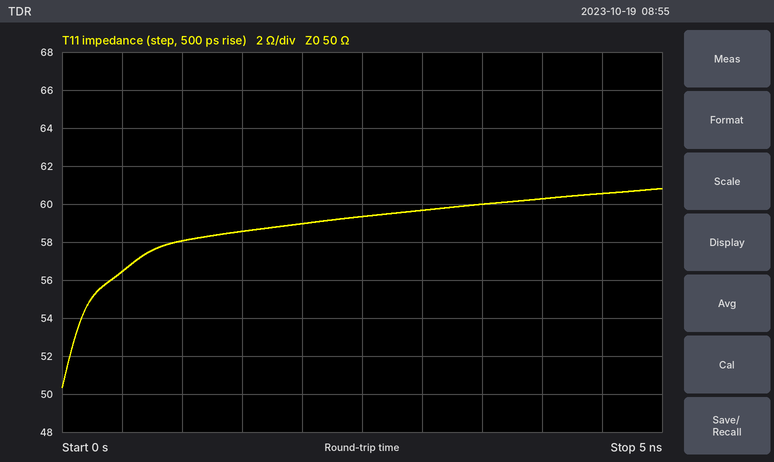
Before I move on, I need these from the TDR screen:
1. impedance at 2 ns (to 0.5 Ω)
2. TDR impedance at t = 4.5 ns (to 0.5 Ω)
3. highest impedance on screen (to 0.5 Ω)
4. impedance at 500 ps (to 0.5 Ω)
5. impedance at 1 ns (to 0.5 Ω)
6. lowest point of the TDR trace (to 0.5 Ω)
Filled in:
59.0 Ω
60.5 Ω
61.0 Ω
56.5 Ω
58.0 Ω
50.5 Ω
